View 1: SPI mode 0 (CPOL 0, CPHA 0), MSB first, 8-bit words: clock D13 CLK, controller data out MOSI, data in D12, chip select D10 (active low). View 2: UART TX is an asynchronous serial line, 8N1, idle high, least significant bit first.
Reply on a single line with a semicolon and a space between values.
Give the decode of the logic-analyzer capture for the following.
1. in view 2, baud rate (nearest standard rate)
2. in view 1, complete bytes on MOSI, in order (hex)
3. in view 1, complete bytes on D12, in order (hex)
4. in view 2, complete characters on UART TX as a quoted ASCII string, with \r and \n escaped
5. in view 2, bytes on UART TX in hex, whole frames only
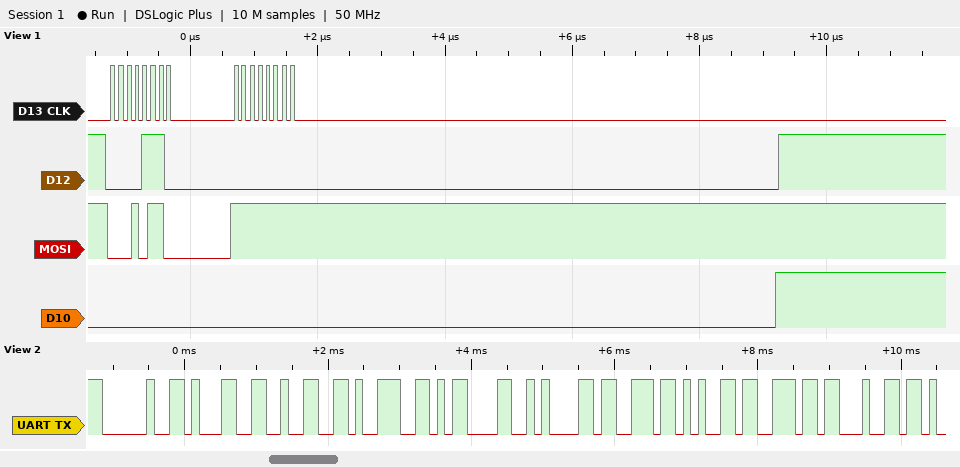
9600 baud; 0x16 0xFF; 0x0E 0x00; " 129\r\nsend"; 20 31 32 39 0D 0A 73 65 6E 64
